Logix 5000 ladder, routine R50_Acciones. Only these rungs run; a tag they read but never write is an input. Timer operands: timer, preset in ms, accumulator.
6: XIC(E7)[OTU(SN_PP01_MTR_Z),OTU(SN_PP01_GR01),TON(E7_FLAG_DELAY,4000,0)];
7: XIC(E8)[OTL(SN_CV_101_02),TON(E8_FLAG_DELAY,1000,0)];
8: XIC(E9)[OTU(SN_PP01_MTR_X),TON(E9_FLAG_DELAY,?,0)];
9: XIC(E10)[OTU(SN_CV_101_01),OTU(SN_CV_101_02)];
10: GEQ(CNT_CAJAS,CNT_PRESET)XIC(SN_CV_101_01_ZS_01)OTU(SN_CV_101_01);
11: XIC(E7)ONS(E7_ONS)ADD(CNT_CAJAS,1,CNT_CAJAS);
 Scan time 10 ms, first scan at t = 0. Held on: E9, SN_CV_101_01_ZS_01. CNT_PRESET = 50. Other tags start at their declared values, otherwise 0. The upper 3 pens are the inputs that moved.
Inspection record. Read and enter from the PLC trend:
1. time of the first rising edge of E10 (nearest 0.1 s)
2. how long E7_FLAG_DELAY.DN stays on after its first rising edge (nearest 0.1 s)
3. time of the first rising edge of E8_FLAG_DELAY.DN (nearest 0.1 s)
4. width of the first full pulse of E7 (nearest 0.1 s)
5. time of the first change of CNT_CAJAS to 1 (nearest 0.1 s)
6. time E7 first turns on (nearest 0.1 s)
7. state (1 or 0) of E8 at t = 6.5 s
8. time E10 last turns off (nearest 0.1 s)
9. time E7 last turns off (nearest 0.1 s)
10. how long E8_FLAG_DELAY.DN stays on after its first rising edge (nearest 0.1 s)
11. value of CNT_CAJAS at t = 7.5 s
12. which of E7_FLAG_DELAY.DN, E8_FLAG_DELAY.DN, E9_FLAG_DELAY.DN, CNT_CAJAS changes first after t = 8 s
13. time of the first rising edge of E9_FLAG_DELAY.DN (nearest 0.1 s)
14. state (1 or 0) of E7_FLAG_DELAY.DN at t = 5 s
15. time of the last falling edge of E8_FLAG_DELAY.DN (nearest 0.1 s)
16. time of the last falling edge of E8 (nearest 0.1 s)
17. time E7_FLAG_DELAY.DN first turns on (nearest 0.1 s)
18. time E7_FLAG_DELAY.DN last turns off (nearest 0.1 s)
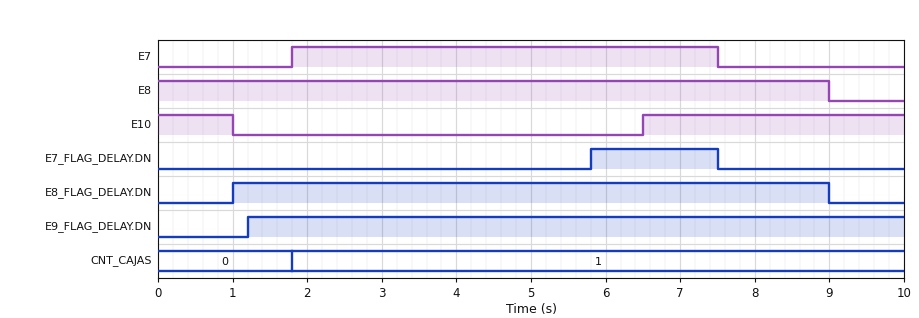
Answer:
6.5 s
1.7 s
1.0 s
5.7 s
1.8 s
1.8 s
1
1.0 s
7.5 s
8.0 s
1
E8_FLAG_DELAY.DN
1.2 s
0
9.0 s
9.0 s
5.8 s
7.5 s
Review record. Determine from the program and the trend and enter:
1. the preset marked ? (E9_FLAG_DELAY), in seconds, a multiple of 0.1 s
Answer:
1.2 s
